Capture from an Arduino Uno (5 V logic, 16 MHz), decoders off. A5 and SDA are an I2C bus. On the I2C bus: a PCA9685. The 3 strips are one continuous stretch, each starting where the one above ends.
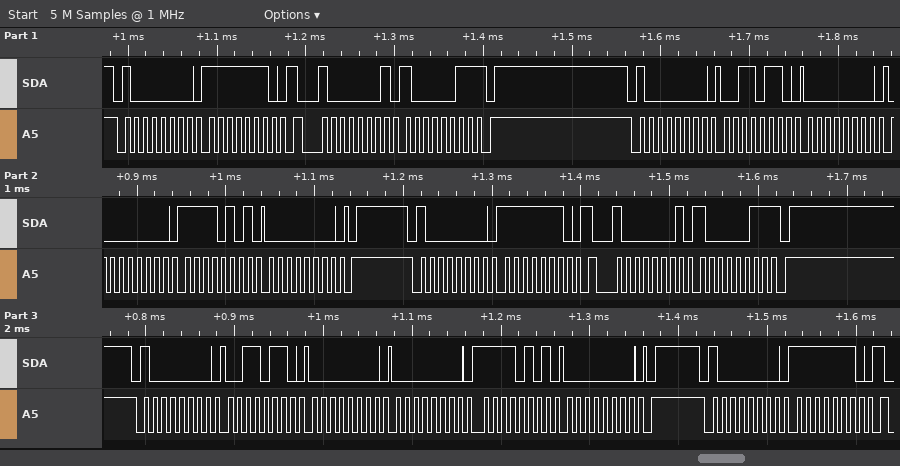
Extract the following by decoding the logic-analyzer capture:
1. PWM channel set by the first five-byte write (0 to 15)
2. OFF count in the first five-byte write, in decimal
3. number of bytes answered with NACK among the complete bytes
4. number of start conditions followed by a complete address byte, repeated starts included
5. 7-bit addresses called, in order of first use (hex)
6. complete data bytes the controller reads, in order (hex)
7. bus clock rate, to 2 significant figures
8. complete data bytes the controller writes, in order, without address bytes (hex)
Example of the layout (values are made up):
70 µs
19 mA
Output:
12
245
2
7
0x40
83 83
100 kHz
FE 36 00 00 F5 00 FE 36 00 00 F5 00 FE
